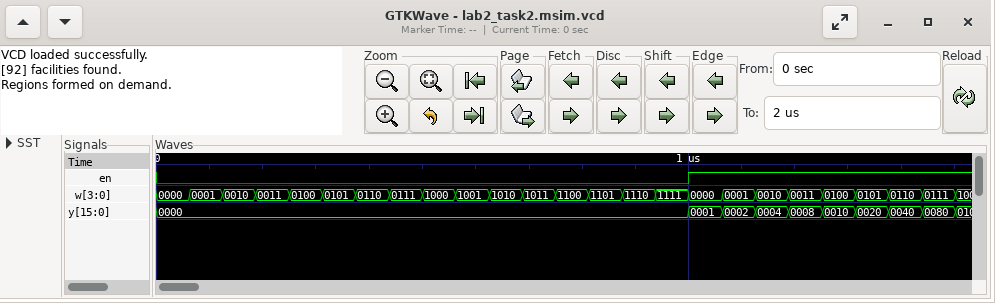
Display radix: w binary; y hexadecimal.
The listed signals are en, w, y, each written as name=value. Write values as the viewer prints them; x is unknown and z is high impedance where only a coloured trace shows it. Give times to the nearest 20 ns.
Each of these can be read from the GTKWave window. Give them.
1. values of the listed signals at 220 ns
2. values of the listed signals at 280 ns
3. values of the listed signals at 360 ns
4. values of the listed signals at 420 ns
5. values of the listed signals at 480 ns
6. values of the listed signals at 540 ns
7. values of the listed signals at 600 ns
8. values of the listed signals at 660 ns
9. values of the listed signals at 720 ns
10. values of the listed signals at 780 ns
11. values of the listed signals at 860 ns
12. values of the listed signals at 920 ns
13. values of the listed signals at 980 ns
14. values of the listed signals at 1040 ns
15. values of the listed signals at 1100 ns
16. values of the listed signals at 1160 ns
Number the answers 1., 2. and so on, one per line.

1. en=0, w=0011, y=0000
2. en=0, w=0100, y=0000
3. en=0, w=0101, y=0000
4. en=0, w=0110, y=0000
5. en=0, w=0111, y=0000
6. en=0, w=1000, y=0000
7. en=0, w=1001, y=0000
8. en=0, w=1010, y=0000
9. en=0, w=1011, y=0000
10. en=0, w=1100, y=0000
11. en=0, w=1101, y=0000
12. en=0, w=1110, y=0000
13. en=0, w=1111, y=0000
14. en=1, w=0000, y=0001
15. en=1, w=0001, y=0002
16. en=1, w=0010, y=0004
